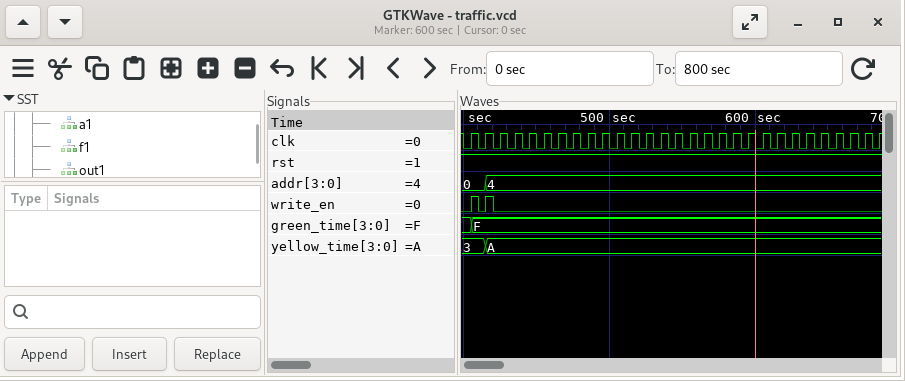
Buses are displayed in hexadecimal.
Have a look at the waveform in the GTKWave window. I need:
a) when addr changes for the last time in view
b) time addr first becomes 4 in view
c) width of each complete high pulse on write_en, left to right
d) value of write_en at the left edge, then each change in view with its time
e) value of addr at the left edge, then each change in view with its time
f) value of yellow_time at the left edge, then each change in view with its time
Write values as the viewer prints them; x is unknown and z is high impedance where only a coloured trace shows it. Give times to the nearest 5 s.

415 s
415 s
5 s, 5 s
0, 1 at 405 s, 0 at 410 s, 1 at 415 s, 0 at 420 s
0, 4 at 415 s
3, A at 415 s
